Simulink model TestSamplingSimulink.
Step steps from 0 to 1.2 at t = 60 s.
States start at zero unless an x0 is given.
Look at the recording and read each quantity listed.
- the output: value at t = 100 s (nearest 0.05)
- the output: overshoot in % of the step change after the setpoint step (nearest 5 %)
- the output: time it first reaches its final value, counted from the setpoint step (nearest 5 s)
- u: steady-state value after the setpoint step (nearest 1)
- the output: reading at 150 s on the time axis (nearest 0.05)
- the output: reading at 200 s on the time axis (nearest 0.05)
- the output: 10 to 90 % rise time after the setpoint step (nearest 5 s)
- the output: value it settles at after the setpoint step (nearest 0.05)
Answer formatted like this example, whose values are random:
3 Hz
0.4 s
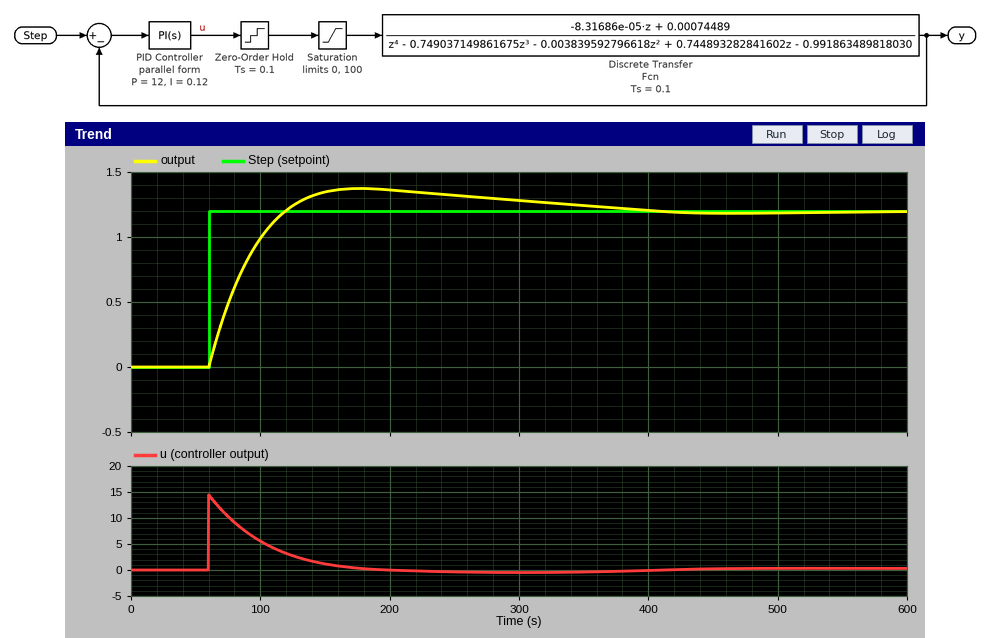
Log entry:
1.00
15 %
60 s
0
1.35
1.35
45 s
1.20
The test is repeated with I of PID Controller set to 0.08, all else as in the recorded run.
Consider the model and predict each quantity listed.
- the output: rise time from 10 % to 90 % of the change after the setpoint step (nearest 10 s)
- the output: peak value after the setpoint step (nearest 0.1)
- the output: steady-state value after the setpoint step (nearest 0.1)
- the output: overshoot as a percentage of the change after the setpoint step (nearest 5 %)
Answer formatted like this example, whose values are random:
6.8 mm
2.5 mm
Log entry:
50 s
1.3
1.2
10 %
